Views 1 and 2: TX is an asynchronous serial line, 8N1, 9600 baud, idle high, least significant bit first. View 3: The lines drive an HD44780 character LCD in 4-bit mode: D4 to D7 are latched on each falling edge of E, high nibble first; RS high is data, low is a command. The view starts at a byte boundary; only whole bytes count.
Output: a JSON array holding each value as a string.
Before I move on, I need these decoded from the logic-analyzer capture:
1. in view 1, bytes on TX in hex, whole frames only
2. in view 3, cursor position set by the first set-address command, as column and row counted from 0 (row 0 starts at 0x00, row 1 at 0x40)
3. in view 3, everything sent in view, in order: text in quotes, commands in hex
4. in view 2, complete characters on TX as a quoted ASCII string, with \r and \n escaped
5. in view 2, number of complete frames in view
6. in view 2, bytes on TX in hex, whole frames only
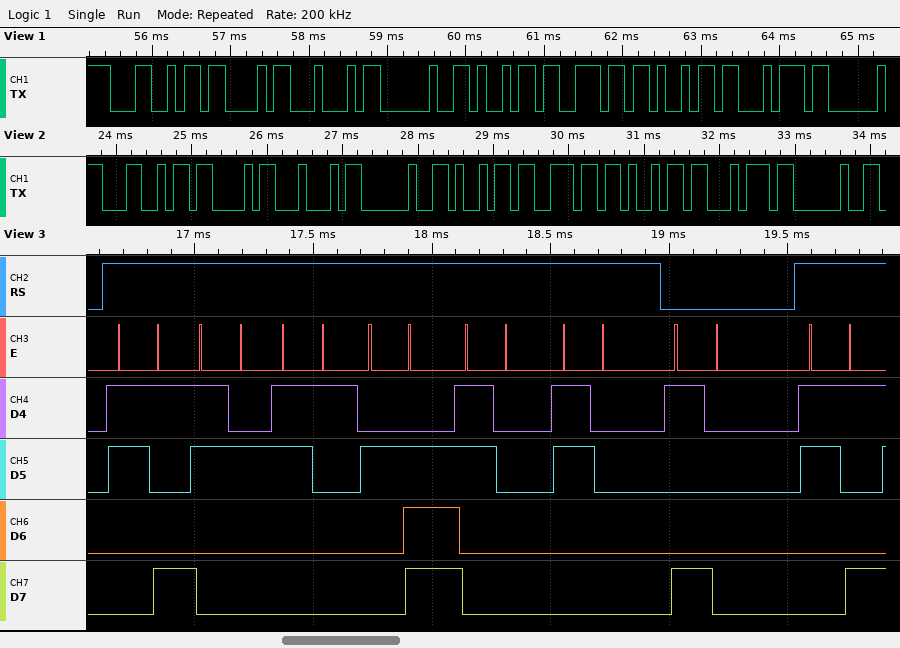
["0x4C 0x43 0x44 0x20 0x69 0x6E 0x69 0x74", "column 16, row 0", "\"921.00\" 0x90 \"9\"", "\"LCD init \"", "9", "4C 43 44 20 69 6E 69 74 20"]
